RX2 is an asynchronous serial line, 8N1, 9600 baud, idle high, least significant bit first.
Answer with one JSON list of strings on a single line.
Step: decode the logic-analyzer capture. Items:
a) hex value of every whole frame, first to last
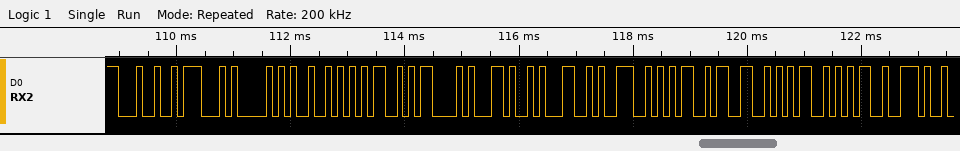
["0x24 0x47 0x50 0x52 0x4D 0x43 0x2C 0x31 0x39 0x35 0x33 0x35 0x35 0x2E"]
